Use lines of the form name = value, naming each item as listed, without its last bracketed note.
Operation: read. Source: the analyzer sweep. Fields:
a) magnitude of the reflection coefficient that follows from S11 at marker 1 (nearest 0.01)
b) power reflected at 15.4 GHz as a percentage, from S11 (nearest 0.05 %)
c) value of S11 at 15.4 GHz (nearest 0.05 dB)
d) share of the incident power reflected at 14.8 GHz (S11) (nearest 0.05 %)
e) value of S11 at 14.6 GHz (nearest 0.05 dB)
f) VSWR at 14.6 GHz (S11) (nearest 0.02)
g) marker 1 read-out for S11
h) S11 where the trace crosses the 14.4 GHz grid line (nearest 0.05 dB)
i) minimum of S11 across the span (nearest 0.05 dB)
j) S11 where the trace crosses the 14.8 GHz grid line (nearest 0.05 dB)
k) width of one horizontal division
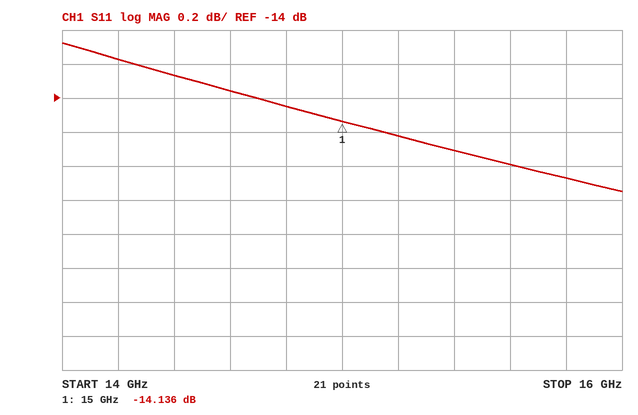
magnitude of the reflection coefficient that follows from S11 at marker 1 = 0.20
power reflected at 15.4 GHz as a percentage, from S11 = 3.70 %
value of S11 at 15.4 GHz = -14.30 dB
share of the incident power reflected at 14.8 GHz (S11) = 3.95 %
value of S11 at 14.6 GHz = -13.95 dB
VSWR at 14.6 GHz (S11) = 1.50
marker 1 read-out for S11 = -14.136 dB
S11 where the trace crosses the 14.4 GHz grid line = -13.85 dB
minimum of S11 across the span = -14.55 dB
S11 where the trace crosses the 14.8 GHz grid line = -14.05 dB
width of one horizontal division = 200 MHz
